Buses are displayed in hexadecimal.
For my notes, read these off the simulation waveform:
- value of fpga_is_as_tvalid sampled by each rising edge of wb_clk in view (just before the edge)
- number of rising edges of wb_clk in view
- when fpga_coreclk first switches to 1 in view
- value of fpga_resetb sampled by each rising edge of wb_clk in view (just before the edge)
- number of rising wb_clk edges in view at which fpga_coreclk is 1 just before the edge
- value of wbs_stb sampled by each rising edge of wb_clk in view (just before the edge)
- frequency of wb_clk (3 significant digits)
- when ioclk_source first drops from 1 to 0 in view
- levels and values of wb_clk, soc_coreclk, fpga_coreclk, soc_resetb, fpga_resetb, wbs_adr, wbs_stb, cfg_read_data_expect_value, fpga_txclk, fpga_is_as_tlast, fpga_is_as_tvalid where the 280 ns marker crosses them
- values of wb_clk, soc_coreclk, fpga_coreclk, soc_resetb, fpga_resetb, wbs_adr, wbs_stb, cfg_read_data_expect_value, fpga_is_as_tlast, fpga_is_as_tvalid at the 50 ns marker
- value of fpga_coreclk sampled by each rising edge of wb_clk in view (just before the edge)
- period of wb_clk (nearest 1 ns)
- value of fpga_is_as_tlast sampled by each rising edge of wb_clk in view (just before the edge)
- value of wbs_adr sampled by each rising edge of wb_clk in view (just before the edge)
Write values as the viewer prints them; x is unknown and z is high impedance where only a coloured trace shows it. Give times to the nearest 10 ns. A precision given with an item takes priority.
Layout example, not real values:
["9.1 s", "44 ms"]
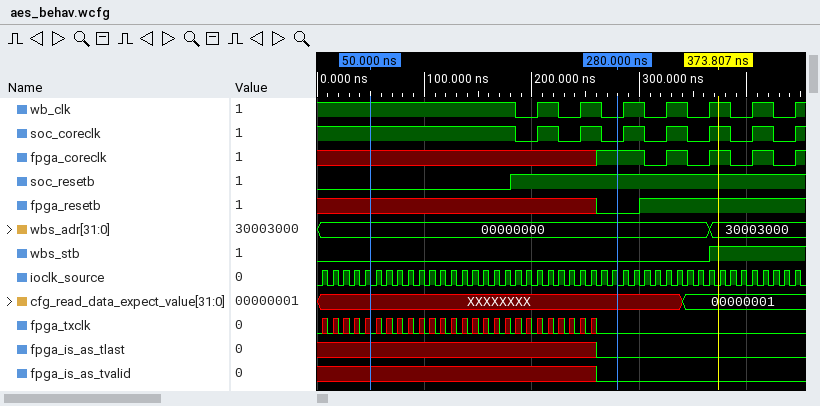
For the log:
["x x 0 0 0 0 0", "7", "260 ns", "x x 0 1 1 1 1", "1", "0 0 0 0 0 1 1", "25.0 MHz", "10 ns", "wb_clk=0, soc_coreclk=0, fpga_coreclk=1, soc_resetb=1, fpga_resetb=0, wbs_adr=00000000, wbs_stb=0, cfg_read_data_expect_value=XXXXXXXX, fpga_txclk=0, fpga_is_as_tlast=0, fpga_is_as_tvalid=0", "wb_clk=1, soc_coreclk=1, fpga_coreclk=x, soc_resetb=0, fpga_resetb=x, wbs_adr=00000000, wbs_stb=0, cfg_read_data_expect_value=XXXXXXXX, fpga_is_as_tlast=x, fpga_is_as_tvalid=x", "x x 1 0 0 0 0", "40 ns", "x x 0 0 0 0 0", "00000000, 00000000, 00000000, 00000000, 00000000, 30003000, 30003000"]
